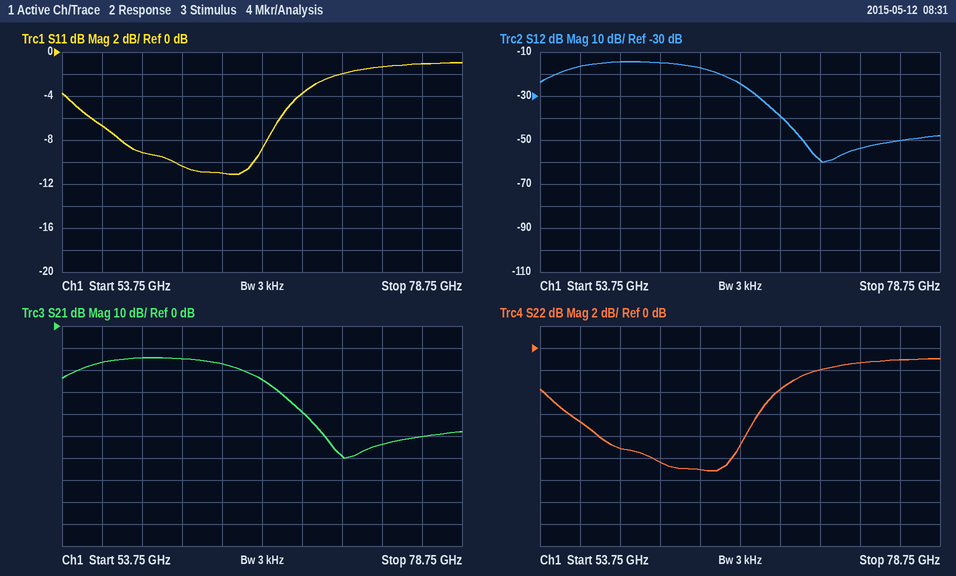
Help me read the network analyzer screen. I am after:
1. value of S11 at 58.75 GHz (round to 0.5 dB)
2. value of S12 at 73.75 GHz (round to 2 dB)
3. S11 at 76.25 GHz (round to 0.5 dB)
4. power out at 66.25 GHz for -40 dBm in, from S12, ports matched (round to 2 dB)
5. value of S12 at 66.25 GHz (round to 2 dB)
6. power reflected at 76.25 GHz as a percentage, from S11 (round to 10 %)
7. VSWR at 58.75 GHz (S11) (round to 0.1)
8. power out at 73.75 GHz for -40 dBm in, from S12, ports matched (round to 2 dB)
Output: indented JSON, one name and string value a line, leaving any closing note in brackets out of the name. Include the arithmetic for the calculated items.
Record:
{
  "value of S11 at 58.75 GHz": "-9.0 dB",
  "value of S12 at 73.75 GHz": "-54 dB",
  "S11 at 76.25 GHz": "-1.0 dB",
  "power out at 66.25 GHz for -40 dBm in, from S12, ports matched": "-40 dBm + (-24 dB) = -64 dBm",
  "value of S12 at 66.25 GHz": "-24 dB",
  "power reflected at 76.25 GHz as a percentage, from S11": "10^(-1/10) ≈ 79.4 %, so 80 % to the nearest 10 %",
  "VSWR at 58.75 GHz (S11)": "|Γ| = 10^(-9/20) = 0.3548; VSWR = (1 + 0.3548)/(1 − 0.3548) ≈ 2.1",
  "power out at 73.75 GHz for -40 dBm in, from S12, ports matched": "-40 dBm + (-54 dB) = -94 dBm"
}
